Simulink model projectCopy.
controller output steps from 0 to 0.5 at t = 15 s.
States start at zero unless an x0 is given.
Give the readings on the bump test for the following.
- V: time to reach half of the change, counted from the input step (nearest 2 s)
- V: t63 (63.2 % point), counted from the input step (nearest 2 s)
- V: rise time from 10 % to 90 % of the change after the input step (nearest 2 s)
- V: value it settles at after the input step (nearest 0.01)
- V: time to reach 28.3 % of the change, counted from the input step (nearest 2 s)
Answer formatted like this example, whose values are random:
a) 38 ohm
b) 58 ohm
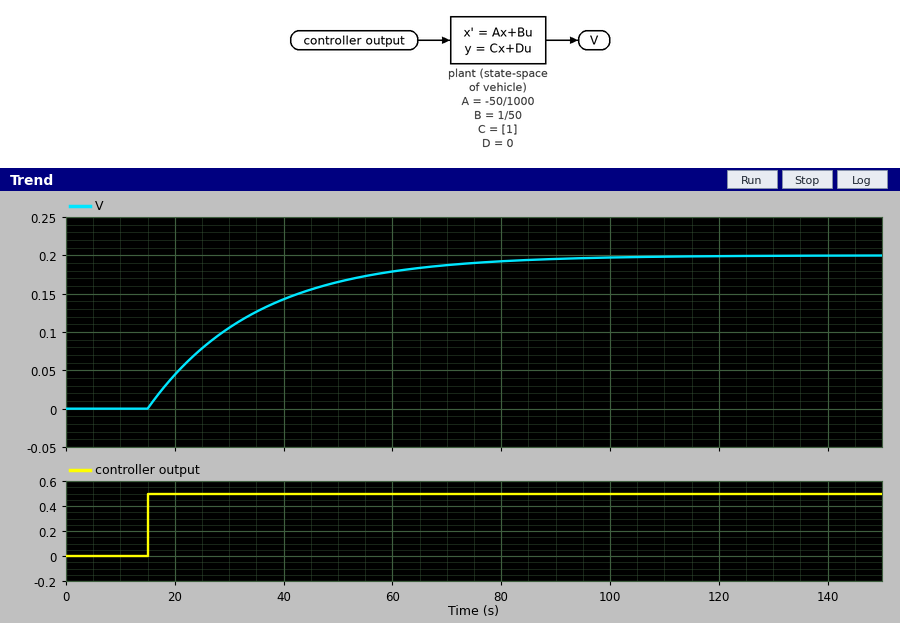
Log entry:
a) 14 s
b) 20 s
c) 44 s
d) 0.20
e) 6 s
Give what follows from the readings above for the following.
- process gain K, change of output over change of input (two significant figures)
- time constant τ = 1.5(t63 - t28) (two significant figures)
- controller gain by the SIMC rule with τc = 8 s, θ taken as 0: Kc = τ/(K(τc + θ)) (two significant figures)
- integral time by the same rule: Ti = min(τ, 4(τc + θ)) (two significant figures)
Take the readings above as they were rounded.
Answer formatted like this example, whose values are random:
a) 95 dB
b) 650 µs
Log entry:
a) 0.40
b) 21 s
c) 6.6
d) 21 s
